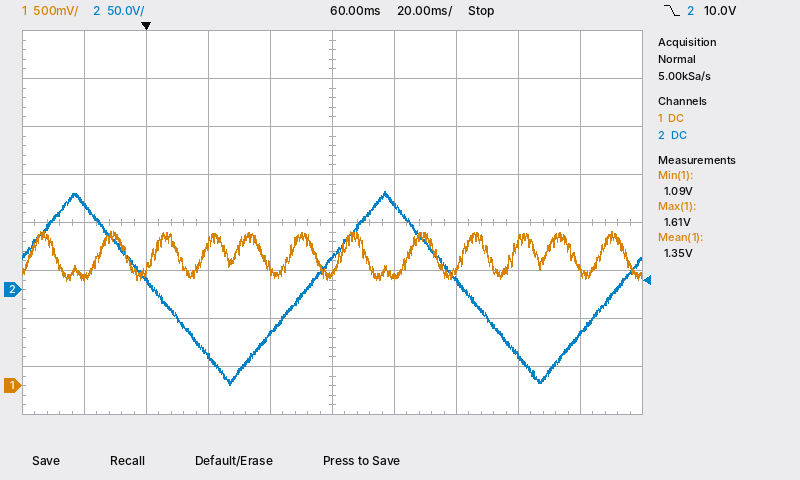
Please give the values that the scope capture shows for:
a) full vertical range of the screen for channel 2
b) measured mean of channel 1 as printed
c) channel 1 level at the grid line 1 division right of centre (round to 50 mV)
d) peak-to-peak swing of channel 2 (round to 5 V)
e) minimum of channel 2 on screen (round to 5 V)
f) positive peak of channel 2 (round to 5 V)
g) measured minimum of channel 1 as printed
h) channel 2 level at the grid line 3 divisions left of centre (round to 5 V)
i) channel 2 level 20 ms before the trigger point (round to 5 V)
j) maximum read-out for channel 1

400 V
1.35 V
1.15 V
200 V
-100 V
100 V
1.09 V
10 V
90 V
1.61 V
